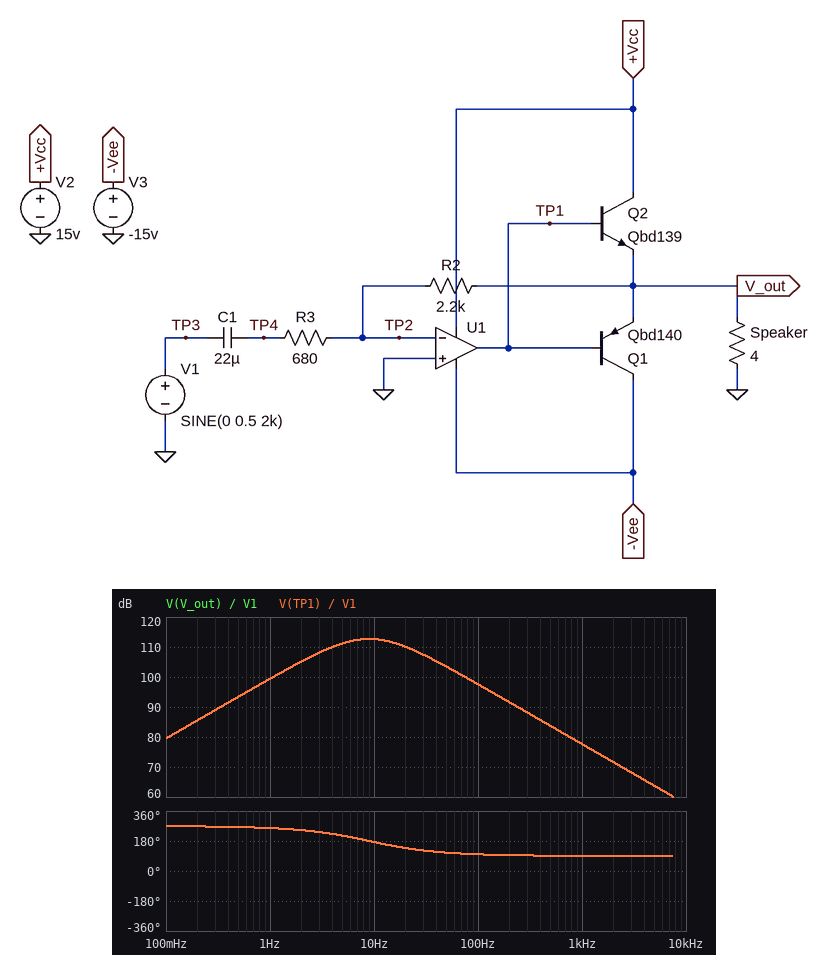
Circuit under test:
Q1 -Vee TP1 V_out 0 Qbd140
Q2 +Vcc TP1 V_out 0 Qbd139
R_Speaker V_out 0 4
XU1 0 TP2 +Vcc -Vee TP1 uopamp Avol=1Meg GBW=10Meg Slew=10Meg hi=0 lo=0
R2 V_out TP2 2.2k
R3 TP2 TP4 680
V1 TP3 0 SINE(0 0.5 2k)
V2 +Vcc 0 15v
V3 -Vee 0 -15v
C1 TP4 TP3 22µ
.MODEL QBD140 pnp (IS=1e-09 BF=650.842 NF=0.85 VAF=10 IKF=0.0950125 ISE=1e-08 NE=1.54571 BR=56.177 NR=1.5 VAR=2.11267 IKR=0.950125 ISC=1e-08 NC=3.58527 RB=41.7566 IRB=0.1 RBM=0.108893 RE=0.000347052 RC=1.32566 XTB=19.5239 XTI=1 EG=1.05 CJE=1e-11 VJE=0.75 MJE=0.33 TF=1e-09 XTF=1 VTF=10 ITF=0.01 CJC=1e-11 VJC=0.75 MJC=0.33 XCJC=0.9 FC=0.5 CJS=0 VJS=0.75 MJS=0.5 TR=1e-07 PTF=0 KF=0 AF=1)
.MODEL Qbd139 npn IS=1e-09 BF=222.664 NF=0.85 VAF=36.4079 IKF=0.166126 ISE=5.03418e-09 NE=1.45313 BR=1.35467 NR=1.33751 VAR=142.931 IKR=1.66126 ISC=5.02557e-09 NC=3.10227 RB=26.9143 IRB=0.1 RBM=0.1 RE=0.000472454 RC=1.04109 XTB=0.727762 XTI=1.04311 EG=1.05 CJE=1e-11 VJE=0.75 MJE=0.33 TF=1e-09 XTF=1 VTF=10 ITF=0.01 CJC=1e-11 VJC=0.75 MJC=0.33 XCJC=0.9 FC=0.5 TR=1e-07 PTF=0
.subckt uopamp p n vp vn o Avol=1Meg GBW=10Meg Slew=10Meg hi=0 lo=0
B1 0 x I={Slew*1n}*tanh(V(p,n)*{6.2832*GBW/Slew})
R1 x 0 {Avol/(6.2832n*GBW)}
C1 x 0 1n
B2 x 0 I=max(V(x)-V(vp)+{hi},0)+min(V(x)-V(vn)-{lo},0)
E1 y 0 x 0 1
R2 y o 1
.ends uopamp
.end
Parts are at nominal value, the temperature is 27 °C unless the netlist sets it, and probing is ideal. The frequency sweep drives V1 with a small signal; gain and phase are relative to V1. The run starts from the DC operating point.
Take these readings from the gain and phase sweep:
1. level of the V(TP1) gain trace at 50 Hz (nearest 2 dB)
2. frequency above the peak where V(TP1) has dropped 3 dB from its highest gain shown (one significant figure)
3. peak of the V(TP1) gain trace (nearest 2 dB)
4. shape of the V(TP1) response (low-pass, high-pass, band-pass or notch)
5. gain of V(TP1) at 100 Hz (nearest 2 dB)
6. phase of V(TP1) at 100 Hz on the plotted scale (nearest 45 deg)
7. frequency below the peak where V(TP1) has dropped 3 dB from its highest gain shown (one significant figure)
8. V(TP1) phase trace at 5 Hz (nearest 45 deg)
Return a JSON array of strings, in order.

["104 dB", "20 Hz", "112 dB", "band-pass", "98 dB", "90 deg", "4 Hz", "225 deg"]
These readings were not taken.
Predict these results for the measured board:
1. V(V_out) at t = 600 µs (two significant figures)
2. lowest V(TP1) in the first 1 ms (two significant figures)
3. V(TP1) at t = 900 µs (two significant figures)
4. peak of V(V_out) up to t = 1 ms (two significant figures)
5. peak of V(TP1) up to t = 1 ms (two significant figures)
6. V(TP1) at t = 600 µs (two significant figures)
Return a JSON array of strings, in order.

["-1.5 V", "-2.1 V", "2.1 V", "1.6 V", "2.2 V", "-2.0 V"]
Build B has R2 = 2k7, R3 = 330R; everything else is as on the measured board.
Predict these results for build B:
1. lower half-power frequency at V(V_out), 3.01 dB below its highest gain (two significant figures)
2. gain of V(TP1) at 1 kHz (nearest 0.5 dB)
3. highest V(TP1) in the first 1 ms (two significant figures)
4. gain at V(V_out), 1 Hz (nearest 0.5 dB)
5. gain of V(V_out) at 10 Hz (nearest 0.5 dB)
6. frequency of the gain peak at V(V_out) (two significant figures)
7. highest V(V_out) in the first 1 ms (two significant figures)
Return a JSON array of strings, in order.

["4.1 Hz", "79.0 dB", "5.1 V", "-12.0 dB", "2.5 dB", "8.8 Hz", "4.1 V"]
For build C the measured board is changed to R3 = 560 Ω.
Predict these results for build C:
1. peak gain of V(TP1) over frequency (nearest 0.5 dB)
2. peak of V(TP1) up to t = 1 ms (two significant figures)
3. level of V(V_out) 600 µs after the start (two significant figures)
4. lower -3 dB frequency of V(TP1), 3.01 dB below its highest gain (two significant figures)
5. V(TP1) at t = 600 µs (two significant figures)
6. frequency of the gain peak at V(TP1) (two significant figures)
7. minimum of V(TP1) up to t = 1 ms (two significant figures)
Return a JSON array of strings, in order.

["113.5 dB", "2.6 V", "-1.9 V", "4.0 Hz", "-2.4 V", "9.2 Hz", "-2.5 V"]
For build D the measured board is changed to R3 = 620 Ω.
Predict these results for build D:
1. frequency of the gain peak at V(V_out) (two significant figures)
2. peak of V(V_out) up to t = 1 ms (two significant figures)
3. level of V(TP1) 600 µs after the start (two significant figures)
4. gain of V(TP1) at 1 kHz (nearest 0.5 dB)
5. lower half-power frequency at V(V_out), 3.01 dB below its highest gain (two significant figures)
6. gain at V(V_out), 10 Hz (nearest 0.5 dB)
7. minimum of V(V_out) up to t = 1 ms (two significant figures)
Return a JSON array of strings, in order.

["9.1 Hz", "1.8 V", "-2.2 V", "78.0 dB", "3.9 Hz", "0 dB", "-1.8 V"]
